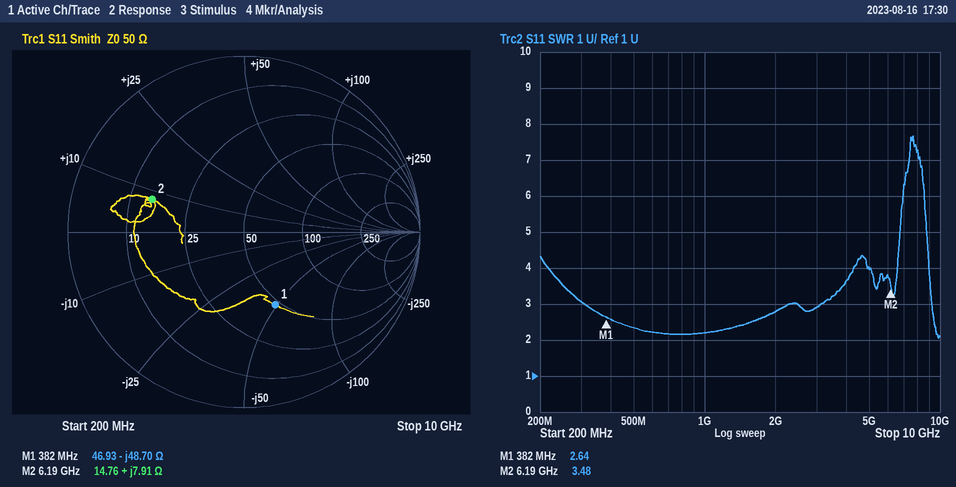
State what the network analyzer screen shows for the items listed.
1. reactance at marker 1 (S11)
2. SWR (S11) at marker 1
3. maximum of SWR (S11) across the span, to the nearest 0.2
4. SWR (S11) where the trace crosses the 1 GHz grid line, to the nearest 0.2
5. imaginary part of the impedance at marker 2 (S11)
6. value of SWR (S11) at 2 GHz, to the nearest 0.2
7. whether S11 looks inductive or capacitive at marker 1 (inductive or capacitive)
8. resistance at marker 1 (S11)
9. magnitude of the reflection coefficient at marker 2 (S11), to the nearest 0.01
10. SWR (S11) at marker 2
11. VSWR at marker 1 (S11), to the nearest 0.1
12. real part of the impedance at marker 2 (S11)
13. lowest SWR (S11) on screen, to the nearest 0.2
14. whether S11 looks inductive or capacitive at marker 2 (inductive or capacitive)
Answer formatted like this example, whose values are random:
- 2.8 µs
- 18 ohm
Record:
- -48.70 Ω
- 2.64
- 7.6
- 2.2
- +7.91 Ω
- 2.8
- capacitive
- 46.93 Ω
- 0.55
- 3.48
- 2.6
- 14.76 Ω
- 2.0
- inductive
